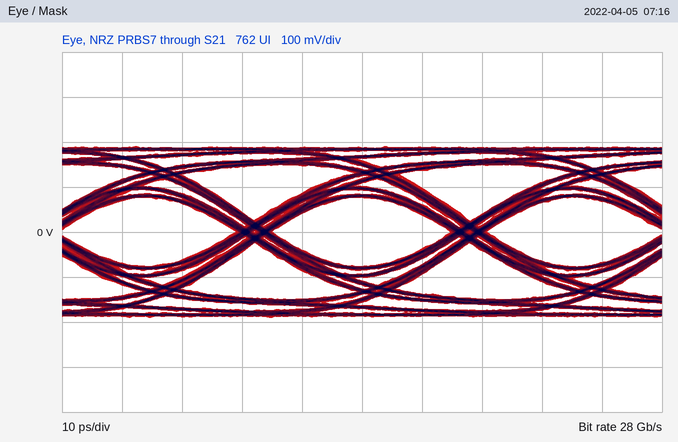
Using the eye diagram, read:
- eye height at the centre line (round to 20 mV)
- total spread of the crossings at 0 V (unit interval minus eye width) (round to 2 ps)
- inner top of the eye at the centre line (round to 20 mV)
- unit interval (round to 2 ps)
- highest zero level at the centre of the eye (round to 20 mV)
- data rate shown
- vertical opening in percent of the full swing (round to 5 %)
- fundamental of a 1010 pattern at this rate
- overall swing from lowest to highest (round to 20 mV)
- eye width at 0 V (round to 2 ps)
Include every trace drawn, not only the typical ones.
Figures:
160 mV
6 ps
80 mV
36 ps
-80 mV
28 Gb/s
40 %
14 GHz
380 mV
30 ps
